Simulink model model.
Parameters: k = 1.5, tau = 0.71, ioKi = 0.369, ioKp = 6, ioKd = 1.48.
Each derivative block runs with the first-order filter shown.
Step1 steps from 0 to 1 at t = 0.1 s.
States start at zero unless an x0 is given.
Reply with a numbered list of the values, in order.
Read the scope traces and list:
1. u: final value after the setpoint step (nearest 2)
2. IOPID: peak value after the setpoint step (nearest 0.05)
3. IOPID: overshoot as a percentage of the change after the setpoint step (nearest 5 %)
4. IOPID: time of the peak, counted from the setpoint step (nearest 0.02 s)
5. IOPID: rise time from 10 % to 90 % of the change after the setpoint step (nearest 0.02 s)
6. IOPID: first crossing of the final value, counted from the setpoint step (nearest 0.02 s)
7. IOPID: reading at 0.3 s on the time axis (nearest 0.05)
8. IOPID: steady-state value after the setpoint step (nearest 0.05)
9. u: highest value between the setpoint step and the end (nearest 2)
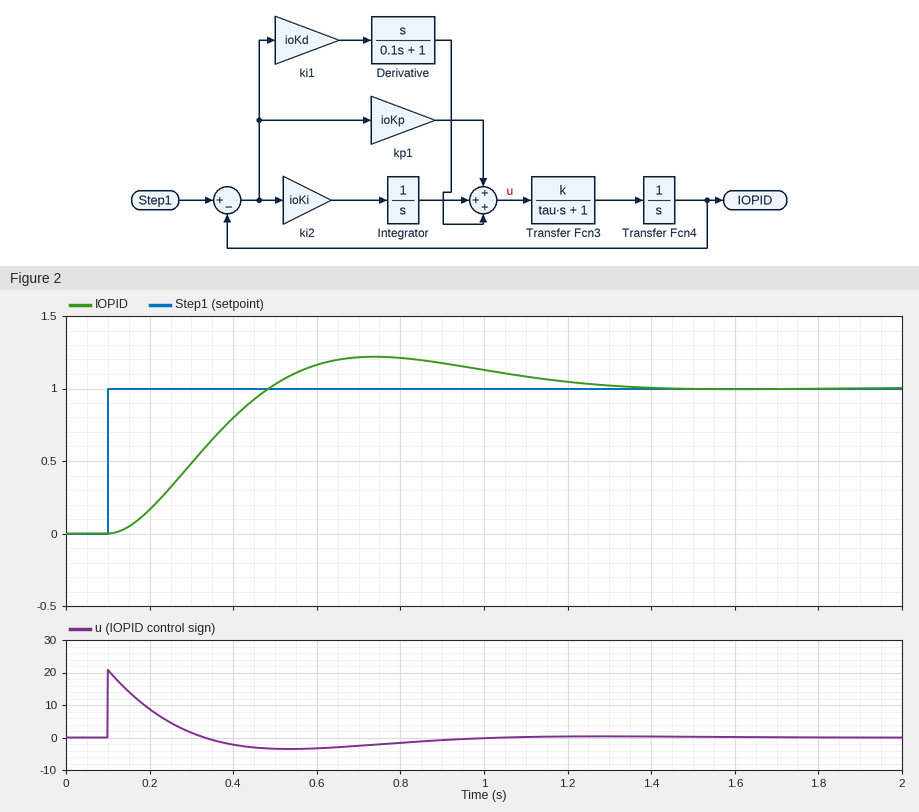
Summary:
1. 0
2. 1.20
3. 20 %
4. 0.64 s
5. 0.26 s
6. 0.38 s
7. 0.50
8. 1.00
9. 20
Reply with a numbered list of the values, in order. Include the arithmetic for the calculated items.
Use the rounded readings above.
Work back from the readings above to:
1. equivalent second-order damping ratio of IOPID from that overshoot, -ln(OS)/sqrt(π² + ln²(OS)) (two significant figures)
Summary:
1. ln(0.2) = -1.609; 1.609 / sqrt(9.870 + 2.590) = 0.46
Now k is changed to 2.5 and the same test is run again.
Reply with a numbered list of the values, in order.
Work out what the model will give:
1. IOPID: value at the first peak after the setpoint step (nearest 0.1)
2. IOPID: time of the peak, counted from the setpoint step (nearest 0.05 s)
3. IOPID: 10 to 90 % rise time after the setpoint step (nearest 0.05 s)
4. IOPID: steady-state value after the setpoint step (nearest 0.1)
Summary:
1. 1.3
2. 0.45 s
3. 0.20 s
4. 1.0
